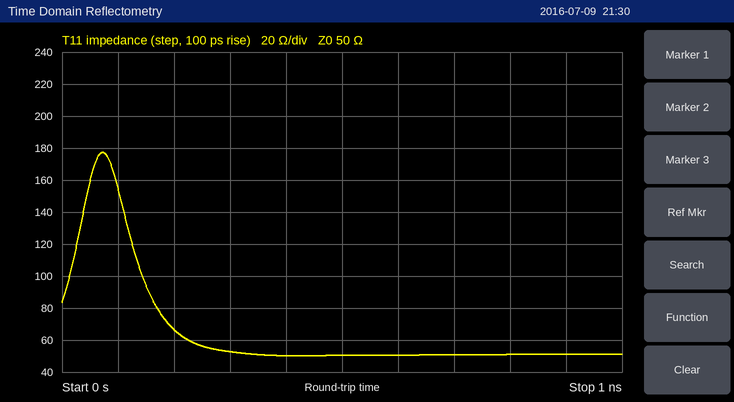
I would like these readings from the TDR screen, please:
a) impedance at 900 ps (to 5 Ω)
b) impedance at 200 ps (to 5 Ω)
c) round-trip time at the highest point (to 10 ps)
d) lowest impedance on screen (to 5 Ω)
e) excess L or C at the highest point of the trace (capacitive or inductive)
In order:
50 Ω
65 Ω
70 ps
50 Ω
inductive
